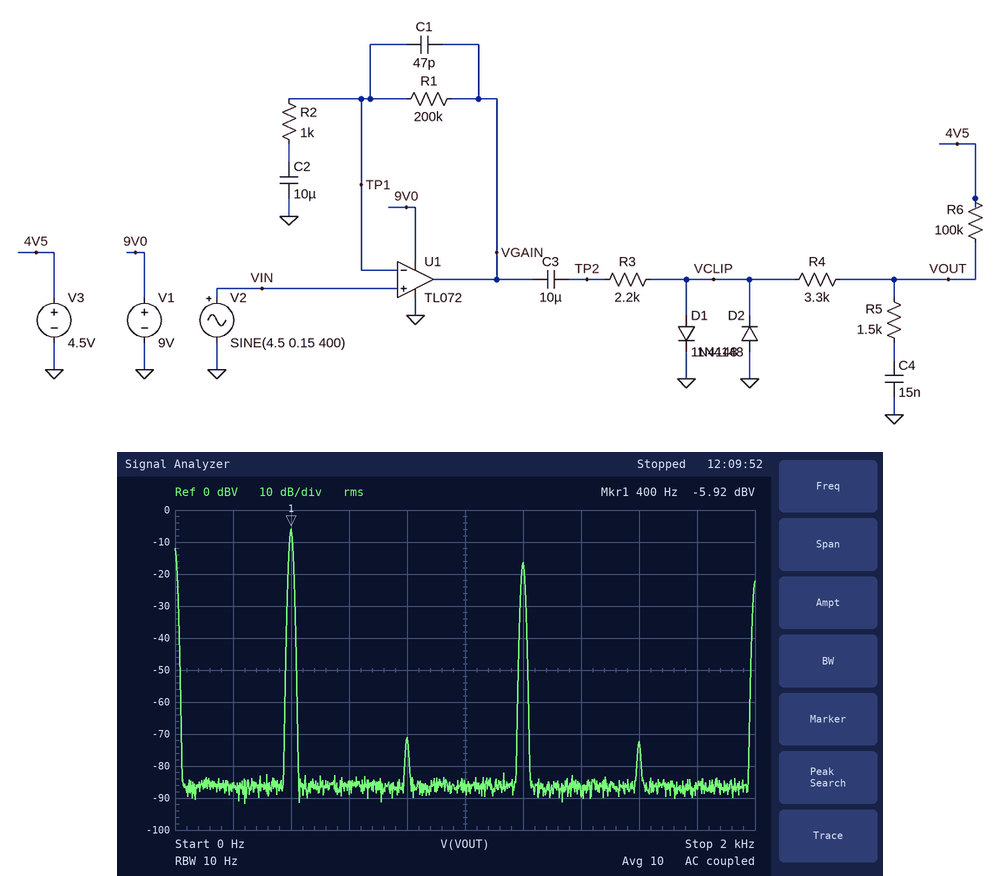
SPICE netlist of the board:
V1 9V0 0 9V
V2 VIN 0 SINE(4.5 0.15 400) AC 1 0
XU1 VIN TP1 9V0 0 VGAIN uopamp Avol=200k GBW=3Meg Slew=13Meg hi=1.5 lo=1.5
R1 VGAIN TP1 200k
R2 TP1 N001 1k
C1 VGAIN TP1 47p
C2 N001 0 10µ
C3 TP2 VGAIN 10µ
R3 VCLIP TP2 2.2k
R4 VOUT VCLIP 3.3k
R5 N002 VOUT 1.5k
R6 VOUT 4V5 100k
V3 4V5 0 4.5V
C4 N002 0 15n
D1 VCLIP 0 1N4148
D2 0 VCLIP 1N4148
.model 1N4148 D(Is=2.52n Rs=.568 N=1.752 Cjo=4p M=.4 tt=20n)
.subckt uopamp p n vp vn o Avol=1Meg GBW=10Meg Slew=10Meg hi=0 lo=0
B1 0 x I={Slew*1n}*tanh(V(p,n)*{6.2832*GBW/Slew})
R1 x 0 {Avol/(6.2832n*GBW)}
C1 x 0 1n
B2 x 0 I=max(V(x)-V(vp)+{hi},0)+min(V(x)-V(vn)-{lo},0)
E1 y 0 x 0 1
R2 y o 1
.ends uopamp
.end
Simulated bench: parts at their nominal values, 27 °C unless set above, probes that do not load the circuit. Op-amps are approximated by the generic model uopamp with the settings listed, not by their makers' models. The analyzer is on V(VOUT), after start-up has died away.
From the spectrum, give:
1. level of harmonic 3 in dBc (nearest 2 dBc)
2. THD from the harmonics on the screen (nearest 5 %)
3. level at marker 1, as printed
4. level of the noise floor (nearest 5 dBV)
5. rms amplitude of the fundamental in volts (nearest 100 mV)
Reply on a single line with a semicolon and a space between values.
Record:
-10 dBc; 30 %; -5.92 dBV; -85 dBV; 500 mV
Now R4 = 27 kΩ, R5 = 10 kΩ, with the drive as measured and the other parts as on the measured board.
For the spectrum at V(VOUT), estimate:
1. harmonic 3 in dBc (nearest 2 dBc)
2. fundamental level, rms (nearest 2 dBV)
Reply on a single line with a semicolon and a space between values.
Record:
-14 dBc; -10 dBV
